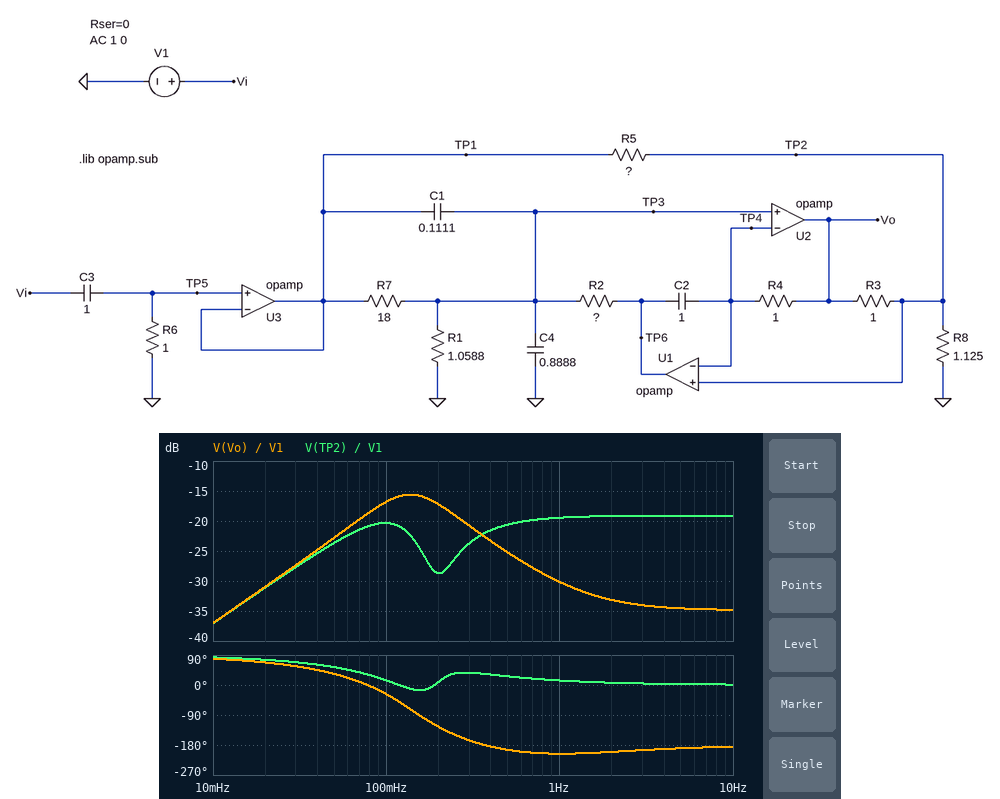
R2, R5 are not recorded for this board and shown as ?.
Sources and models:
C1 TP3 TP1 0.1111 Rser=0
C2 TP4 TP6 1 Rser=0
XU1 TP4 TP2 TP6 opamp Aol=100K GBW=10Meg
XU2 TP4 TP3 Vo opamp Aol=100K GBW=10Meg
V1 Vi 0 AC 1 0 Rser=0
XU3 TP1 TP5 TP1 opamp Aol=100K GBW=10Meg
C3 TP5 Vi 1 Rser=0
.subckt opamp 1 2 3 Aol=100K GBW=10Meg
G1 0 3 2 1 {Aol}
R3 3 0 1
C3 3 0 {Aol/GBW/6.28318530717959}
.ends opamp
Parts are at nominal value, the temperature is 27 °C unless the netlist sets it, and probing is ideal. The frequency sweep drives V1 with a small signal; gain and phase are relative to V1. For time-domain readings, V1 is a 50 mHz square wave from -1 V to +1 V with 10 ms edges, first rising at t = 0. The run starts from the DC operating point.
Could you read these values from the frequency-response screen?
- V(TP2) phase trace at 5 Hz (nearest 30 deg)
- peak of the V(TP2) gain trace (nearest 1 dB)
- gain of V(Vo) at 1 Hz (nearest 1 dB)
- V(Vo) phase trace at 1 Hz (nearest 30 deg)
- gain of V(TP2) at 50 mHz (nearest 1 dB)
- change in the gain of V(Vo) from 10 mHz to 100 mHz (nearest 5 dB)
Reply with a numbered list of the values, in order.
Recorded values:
1. 0 deg
2. -19 dB
3. -30 dB
4. -210 deg
5. -24 dB
6. 20 dB
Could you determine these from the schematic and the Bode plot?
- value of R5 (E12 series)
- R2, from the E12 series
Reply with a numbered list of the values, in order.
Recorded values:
1. 3.9 Ω
2. 1.5 Ω
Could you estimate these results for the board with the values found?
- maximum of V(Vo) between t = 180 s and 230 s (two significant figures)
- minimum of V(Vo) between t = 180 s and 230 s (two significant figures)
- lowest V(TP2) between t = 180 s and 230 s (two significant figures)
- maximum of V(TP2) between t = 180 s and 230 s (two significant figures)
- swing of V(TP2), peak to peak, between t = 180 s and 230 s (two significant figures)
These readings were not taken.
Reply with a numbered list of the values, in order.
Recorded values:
1. 180 mV
2. -180 mV
3. -220 mV
4. 220 mV
5. 440 mV
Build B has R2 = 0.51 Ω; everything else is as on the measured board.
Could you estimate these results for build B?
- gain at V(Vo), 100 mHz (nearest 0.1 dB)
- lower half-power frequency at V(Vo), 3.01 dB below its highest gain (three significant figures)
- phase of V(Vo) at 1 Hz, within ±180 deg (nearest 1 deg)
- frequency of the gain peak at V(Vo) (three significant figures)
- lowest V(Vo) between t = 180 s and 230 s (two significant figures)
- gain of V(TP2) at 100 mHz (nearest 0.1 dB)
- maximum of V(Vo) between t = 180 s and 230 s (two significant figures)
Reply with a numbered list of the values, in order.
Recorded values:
1. -17.0 dB
2. 155 mHz
3. 163 deg
4. 227 mHz
5. -300 mV
6. -18.0 dB
7. 300 mV
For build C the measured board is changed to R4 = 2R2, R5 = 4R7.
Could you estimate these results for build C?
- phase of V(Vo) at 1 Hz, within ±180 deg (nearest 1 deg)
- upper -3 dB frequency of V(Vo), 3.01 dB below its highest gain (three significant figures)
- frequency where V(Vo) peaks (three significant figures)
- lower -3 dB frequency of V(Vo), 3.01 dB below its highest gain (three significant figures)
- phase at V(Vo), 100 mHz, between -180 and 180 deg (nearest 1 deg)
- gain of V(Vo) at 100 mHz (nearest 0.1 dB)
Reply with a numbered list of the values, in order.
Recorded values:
1. 57 deg
2. 242 mHz
3. 100 mHz
4. 45.2 mHz
5. -85 deg
6. -23.2 dB
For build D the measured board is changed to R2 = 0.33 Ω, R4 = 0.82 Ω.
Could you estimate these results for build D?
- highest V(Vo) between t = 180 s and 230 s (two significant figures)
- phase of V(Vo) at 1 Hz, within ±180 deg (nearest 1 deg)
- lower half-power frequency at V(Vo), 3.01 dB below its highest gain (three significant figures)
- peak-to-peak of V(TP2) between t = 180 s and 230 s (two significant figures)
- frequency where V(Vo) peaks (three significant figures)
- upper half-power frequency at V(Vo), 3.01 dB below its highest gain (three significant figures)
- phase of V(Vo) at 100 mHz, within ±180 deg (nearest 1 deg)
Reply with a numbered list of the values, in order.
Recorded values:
1. 380 mV
2. 172 deg
3. 236 mHz
4. 490 mV
5. 316 mHz
6. 393 mHz
7. 43 deg
